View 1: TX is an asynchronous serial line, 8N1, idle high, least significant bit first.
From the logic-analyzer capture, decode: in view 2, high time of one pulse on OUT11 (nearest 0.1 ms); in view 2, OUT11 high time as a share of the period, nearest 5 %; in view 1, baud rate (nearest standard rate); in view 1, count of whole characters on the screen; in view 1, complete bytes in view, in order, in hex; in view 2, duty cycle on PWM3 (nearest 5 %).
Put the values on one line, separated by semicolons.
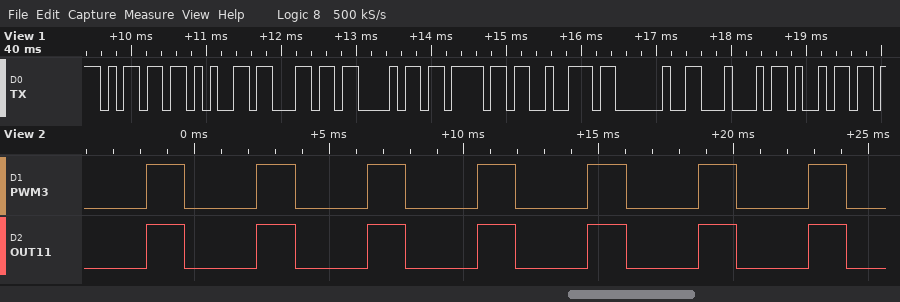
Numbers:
1.4 ms; 35 %; 9600 baud; 9; 6D 65 6C 68 6F 72 20 44 69; 35 %
